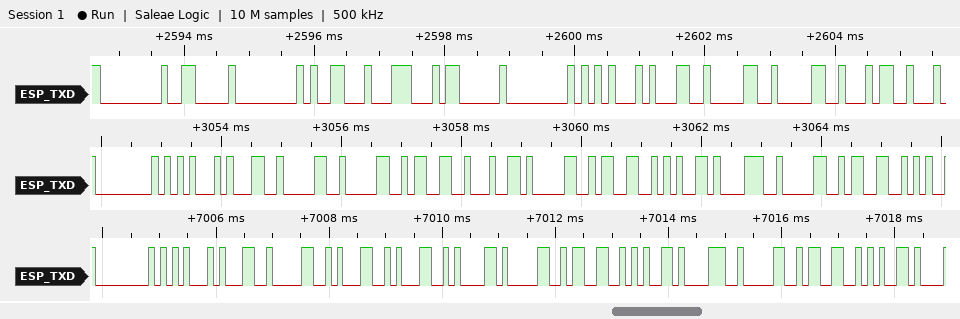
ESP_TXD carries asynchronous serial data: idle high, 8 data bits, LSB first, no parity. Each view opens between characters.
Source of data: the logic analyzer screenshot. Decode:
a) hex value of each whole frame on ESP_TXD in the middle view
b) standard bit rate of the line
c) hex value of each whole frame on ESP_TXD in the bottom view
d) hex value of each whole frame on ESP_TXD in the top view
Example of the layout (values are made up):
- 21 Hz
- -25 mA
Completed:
- 00, 15, 31, 30, 30, 33, 64, 30, 33, 65, 38, 30, 33
- 9600 baud
- 00, 15, 31, 30, 31, 31, 61, 30, 33, 65, 38, 30, 33, 65
- 00, 06, 00, 19, 1C, 03, 00, 15, 31, 30, 30, 34
